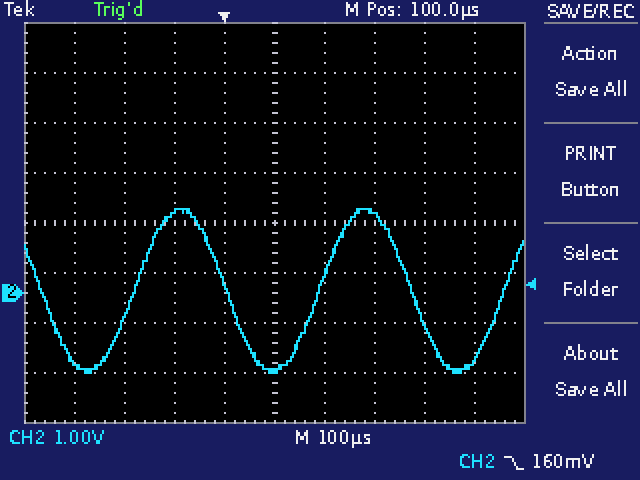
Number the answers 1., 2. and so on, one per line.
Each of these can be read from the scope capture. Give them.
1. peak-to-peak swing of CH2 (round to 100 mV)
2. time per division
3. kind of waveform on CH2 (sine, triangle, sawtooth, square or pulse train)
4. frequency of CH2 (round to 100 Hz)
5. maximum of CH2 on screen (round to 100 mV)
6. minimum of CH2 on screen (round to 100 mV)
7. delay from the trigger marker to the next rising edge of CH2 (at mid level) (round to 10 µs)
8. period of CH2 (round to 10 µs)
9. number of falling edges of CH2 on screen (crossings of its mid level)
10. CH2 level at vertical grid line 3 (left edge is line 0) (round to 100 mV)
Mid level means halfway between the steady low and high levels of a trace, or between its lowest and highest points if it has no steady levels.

1. 3.3 V
2. 100 µs
3. sine
4. 2.7 kHz
5. 1.7 V
6. -1.6 V
7. 190 µs
8. 370 µs
9. 3
10. 1.6 V
